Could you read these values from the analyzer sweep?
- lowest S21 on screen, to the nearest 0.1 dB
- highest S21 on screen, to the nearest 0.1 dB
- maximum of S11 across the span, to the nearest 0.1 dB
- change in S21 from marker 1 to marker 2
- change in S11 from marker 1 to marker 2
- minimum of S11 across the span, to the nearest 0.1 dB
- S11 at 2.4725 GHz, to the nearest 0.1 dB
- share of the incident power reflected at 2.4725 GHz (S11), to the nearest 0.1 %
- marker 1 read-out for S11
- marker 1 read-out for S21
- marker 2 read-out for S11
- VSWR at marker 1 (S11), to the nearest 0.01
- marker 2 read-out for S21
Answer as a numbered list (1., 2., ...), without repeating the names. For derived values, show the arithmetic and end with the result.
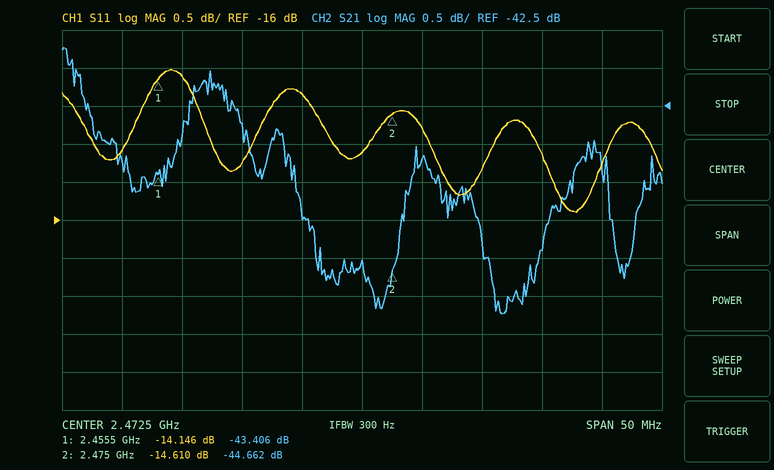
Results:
1. -45.2 dB
2. -41.7 dB
3. -14.0 dB
4. -44.662 − (-43.406) = -1.256 dB
5. -14.61 − (-14.146) = -0.464 dB
6. -15.9 dB
7. -15.1 dB
8. 10^(-15.1/10) ≈ 3.1 %
9. -14.146 dB
10. -43.406 dB
11. -14.610 dB
12. (1 + 0.1962)/(1 − 0.1962) ≈ 1.49
13. -44.662 dB
